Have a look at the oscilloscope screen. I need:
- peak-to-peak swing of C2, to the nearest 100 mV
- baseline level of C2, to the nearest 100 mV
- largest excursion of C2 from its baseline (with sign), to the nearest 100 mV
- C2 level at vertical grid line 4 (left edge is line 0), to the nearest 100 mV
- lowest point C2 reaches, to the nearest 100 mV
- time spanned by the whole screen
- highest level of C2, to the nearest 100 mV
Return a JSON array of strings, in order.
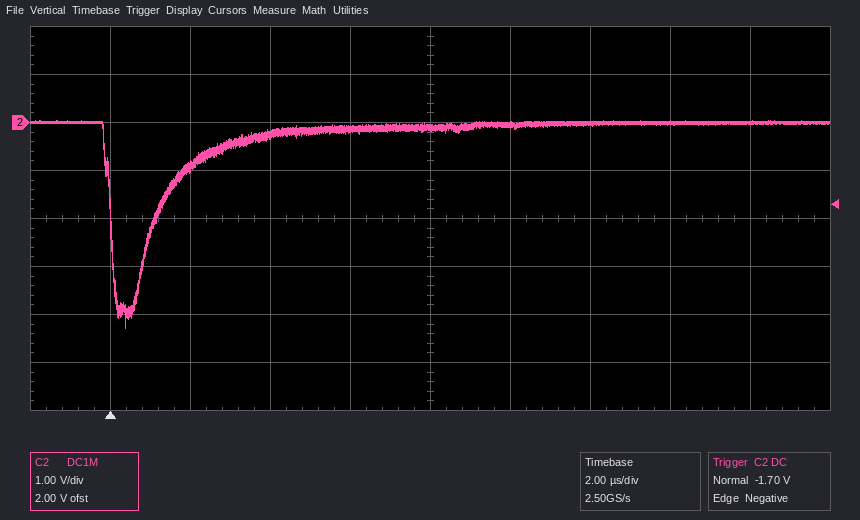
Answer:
["4.3 V", "0.0 V", "-4.3 V", "-100 mV", "-4.3 V", "20 µs", "0.0 V"]
